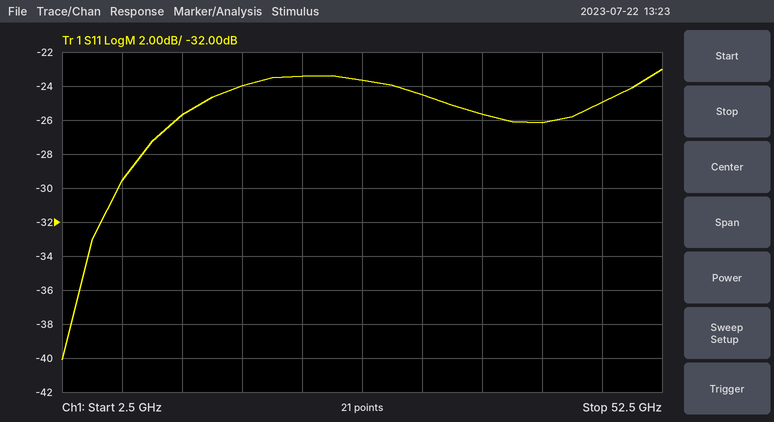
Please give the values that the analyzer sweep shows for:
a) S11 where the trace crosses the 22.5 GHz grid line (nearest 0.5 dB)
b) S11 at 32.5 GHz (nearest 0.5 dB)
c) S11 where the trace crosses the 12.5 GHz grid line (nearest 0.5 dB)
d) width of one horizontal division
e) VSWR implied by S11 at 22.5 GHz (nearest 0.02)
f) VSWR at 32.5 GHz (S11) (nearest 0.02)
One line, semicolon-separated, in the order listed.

-23.5 dB; -24.5 dB; -25.5 dB; 5 GHz; 1.14; 1.12
